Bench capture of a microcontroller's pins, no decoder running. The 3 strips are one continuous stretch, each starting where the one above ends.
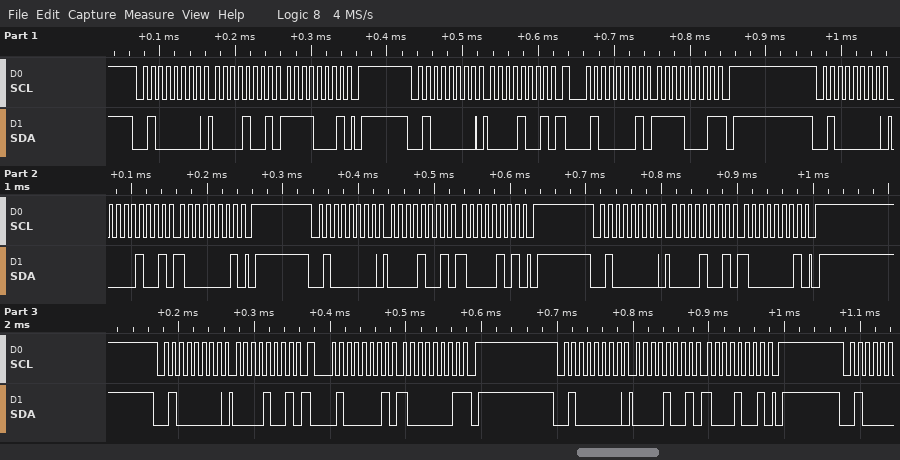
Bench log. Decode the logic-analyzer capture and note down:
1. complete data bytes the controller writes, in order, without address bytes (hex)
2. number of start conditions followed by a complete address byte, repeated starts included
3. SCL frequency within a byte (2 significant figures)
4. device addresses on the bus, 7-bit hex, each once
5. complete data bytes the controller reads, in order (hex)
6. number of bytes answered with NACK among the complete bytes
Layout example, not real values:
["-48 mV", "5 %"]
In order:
["09 F1 09 09 81 09 85 09 81 09 09 89", "9", "100 kHz", "0x20", "F1 81", "2"]
